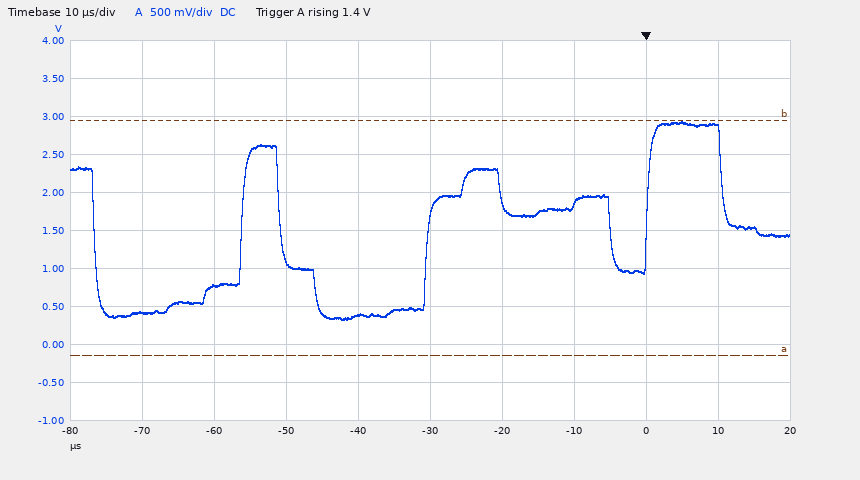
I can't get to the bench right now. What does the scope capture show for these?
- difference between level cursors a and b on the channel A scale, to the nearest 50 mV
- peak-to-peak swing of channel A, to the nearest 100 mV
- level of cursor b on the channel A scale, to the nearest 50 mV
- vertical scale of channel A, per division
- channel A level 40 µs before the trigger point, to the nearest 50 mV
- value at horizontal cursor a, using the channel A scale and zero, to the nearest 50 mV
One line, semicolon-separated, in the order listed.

3.10 V; 2.60 V; 2.95 V; 500 mV; 400 mV; -150 mV
